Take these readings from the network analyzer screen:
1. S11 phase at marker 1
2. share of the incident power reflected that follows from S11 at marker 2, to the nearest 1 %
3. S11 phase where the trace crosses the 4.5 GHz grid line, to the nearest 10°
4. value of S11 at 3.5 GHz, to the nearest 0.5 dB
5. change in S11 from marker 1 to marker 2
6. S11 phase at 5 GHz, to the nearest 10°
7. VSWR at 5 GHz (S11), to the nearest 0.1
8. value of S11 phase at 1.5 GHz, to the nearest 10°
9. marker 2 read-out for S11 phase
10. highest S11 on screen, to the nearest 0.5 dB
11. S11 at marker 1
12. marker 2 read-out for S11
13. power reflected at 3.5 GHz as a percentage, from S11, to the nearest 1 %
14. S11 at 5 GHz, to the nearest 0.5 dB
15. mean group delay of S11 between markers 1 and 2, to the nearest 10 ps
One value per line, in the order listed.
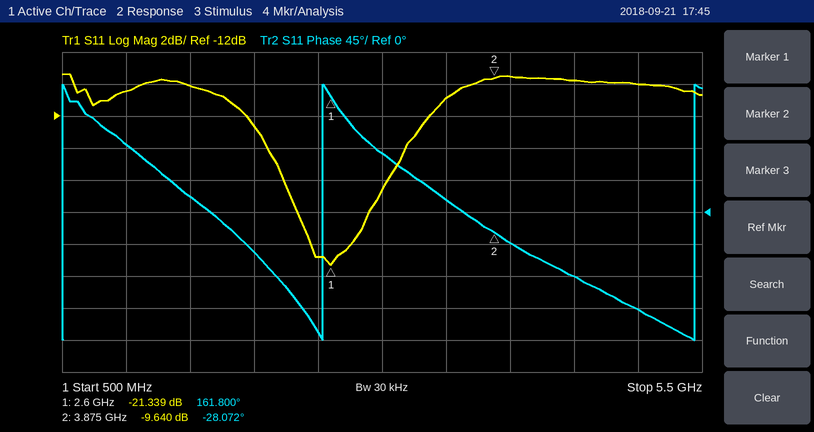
161.800°
11 %
-90°
-11.0 dB
11.699 dB
-140°
1.9
20°
-28.072°
-9.5 dB
-21.339 dB
-9.640 dB
8 %
-10.0 dB
410 ps
